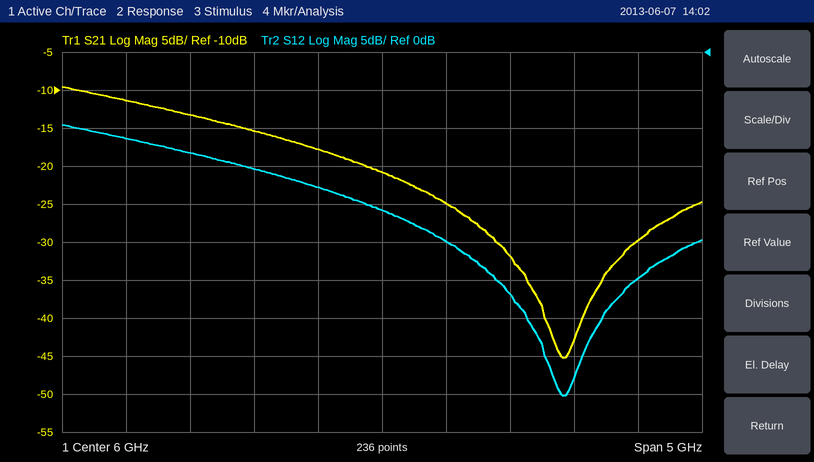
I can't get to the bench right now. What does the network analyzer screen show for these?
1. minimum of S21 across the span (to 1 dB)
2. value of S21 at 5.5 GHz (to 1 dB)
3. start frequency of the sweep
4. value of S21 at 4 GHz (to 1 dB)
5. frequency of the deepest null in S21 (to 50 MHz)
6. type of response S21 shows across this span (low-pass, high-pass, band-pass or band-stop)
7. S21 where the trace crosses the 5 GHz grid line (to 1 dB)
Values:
-45 dB
-18 dB
3.5 GHz
-11 dB
7.40 GHz
low-pass
-15 dB
